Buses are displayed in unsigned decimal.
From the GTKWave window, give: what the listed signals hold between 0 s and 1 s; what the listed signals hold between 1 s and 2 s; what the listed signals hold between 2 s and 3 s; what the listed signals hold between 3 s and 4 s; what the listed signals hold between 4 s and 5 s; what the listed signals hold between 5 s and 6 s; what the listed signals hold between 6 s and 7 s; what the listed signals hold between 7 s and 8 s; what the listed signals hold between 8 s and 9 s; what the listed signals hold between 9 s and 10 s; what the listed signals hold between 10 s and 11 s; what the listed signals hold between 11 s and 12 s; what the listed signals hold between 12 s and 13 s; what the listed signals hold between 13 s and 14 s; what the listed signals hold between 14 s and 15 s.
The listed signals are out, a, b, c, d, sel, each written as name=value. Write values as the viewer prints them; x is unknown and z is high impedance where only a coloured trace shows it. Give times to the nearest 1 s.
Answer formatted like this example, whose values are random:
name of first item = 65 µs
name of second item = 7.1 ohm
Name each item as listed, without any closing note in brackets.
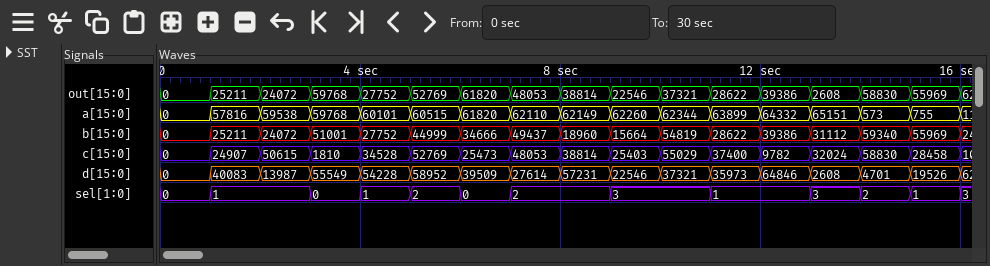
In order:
what the listed signals hold between 0 s and 1 s = out=0, a=0, b=0, c=0, d=0, sel=0
what the listed signals hold between 1 s and 2 s = out=25211, a=57816, b=25211, c=24907, d=40083, sel=1
what the listed signals hold between 2 s and 3 s = out=24072, a=59538, b=24072, c=50615, d=13987, sel=1
what the listed signals hold between 3 s and 4 s = out=59768, a=59768, b=51001, c=1810, d=55549, sel=0
what the listed signals hold between 4 s and 5 s = out=27752, a=60101, b=27752, c=34528, d=54228, sel=1
what the listed signals hold between 5 s and 6 s = out=52769, a=60515, b=44999, c=52769, d=58952, sel=2
what the listed signals hold between 6 s and 7 s = out=61820, a=61820, b=34666, c=25473, d=39509, sel=0
what the listed signals hold between 7 s and 8 s = out=48053, a=62110, b=49437, c=48053, d=27614, sel=2
what the listed signals hold between 8 s and 9 s = out=38814, a=62149, b=18960, c=38814, d=57231, sel=2
what the listed signals hold between 9 s and 10 s = out=22546, a=62260, b=15664, c=25403, d=22546, sel=3
what the listed signals hold between 10 s and 11 s = out=37321, a=62344, b=54819, c=55029, d=37321, sel=3
what the listed signals hold between 11 s and 12 s = out=28622, a=63899, b=28622, c=37400, d=35973, sel=1
what the listed signals hold between 12 s and 13 s = out=39386, a=64332, b=39386, c=9782, d=64846, sel=1
what the listed signals hold between 13 s and 14 s = out=2608, a=65151, b=31112, c=32024, d=2608, sel=3
what the listed signals hold between 14 s and 15 s = out=58830, a=573, b=59340, c=58830, d=4701, sel=2
